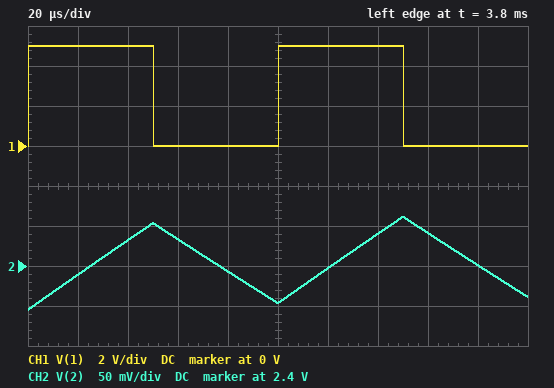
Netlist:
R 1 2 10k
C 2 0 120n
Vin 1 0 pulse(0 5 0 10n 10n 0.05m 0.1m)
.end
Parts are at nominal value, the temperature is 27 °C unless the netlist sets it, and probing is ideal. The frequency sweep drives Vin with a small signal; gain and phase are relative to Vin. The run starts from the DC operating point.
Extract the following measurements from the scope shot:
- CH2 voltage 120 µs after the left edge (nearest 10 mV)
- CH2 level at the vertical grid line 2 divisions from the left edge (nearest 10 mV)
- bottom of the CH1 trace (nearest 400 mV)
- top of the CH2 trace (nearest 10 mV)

2.40 V
2.43 V
0 V
2.46 V
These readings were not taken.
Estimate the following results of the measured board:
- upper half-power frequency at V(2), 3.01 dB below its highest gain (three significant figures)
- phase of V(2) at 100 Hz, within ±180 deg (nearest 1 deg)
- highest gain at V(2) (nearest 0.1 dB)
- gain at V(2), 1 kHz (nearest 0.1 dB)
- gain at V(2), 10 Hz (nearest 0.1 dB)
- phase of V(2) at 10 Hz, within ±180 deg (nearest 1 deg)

133 Hz
-37 deg
0 dB
-17.6 dB
0 dB
-4 deg
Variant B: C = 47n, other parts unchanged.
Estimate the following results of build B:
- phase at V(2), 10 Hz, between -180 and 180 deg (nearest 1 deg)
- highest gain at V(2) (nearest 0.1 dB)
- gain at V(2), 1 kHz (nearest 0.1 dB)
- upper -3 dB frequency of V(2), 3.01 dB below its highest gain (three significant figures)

-2 deg
0 dB
-9.9 dB
339 Hz
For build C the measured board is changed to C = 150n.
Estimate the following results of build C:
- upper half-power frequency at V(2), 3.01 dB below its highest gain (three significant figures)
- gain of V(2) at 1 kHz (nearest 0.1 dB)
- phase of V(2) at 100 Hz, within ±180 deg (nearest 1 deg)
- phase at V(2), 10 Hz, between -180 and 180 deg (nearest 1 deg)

106 Hz
-19.5 dB
-43 deg
-5 deg
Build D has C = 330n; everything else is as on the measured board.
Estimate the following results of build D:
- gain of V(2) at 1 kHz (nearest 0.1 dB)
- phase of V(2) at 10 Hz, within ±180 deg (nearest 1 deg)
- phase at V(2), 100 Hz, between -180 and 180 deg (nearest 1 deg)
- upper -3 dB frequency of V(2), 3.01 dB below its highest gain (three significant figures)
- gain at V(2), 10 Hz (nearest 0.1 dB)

-26.3 dB
-12 deg
-64 deg
48.2 Hz
-0.2 dB
